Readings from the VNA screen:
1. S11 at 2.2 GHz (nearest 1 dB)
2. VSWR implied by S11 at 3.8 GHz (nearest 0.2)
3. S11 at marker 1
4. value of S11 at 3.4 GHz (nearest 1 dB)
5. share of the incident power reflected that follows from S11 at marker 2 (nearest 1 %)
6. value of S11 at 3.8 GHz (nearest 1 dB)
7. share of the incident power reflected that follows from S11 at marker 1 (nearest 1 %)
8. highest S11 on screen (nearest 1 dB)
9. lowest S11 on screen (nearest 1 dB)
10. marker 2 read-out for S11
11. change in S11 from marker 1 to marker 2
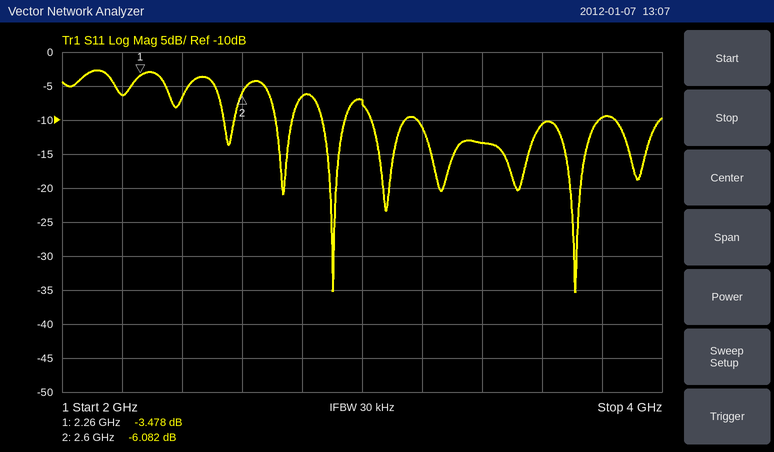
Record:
-6 dB
2.0
-3.478 dB
-13 dB
25 %
-10 dB
45 %
-3 dB
-35 dB
-6.082 dB
-2.604 dB
